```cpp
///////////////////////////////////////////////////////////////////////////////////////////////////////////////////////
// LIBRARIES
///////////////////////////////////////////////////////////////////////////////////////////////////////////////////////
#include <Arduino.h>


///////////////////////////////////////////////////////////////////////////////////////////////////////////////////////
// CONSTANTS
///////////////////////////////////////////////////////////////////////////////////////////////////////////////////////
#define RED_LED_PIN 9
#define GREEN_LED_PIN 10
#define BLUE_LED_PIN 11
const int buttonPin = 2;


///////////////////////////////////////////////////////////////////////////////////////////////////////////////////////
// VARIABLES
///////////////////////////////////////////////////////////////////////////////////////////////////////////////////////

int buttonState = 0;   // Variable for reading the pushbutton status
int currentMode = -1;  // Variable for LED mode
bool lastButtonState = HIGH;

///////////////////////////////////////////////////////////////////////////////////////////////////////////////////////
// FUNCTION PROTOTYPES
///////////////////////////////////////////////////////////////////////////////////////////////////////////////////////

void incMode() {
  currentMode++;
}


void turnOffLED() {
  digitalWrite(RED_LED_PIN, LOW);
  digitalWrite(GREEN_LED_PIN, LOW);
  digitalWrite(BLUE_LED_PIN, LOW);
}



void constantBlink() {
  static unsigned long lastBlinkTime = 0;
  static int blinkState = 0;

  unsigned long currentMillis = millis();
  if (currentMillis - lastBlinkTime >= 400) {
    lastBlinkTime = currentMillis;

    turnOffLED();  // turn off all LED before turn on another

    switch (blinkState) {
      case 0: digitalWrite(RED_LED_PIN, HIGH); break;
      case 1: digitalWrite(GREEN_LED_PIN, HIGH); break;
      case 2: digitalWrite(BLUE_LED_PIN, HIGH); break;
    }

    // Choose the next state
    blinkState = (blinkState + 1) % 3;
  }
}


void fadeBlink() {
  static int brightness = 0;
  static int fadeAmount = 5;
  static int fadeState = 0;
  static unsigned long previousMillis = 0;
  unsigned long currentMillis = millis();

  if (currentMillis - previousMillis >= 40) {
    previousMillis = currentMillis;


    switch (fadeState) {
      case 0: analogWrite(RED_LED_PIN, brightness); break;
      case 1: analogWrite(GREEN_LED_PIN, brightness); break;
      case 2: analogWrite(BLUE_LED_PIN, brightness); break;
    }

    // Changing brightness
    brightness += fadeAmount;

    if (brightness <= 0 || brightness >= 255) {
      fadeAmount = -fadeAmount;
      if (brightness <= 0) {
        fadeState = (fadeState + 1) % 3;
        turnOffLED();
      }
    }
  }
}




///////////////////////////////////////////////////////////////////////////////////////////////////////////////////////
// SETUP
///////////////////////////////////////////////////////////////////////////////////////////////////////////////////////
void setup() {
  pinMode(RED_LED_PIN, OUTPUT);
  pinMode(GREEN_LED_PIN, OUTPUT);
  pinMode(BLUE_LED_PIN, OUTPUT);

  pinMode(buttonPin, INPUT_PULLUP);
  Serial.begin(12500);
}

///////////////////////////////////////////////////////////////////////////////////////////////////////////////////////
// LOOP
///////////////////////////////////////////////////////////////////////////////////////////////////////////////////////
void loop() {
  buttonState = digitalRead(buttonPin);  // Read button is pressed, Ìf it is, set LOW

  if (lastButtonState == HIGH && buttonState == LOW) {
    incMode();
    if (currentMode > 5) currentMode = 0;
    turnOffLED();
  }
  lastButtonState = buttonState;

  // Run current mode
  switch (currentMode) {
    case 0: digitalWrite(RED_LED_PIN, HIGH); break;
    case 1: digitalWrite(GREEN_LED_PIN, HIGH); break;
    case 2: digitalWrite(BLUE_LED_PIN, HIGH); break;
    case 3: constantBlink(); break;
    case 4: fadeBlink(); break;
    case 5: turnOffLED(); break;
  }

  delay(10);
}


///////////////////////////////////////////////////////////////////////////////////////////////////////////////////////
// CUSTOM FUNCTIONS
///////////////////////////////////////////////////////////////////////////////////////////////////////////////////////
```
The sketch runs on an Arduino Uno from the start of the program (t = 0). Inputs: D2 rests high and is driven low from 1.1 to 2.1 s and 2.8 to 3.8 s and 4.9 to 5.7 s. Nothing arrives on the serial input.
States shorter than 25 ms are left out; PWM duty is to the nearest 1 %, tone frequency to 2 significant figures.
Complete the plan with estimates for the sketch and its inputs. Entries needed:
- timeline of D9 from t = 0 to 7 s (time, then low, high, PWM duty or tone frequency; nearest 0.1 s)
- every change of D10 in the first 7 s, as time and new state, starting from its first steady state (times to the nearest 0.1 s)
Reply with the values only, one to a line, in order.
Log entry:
0 s low; 1.1 s high; 2.8 s low
0 s low; 2.8 s high; 4.9 s low
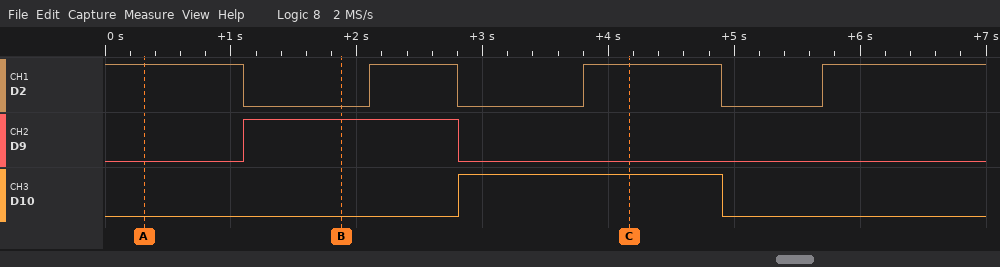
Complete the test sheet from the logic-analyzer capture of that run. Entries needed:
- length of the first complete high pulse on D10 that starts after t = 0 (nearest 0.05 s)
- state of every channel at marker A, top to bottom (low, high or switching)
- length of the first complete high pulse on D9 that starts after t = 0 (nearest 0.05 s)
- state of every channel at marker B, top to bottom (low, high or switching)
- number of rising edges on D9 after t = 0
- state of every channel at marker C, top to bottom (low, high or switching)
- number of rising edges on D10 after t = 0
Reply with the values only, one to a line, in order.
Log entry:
2.10 s
D2 high, D9 low, D10 low
1.70 s
D2 low, D9 high, D10 low
1
D2 high, D9 low, D10 high
1
